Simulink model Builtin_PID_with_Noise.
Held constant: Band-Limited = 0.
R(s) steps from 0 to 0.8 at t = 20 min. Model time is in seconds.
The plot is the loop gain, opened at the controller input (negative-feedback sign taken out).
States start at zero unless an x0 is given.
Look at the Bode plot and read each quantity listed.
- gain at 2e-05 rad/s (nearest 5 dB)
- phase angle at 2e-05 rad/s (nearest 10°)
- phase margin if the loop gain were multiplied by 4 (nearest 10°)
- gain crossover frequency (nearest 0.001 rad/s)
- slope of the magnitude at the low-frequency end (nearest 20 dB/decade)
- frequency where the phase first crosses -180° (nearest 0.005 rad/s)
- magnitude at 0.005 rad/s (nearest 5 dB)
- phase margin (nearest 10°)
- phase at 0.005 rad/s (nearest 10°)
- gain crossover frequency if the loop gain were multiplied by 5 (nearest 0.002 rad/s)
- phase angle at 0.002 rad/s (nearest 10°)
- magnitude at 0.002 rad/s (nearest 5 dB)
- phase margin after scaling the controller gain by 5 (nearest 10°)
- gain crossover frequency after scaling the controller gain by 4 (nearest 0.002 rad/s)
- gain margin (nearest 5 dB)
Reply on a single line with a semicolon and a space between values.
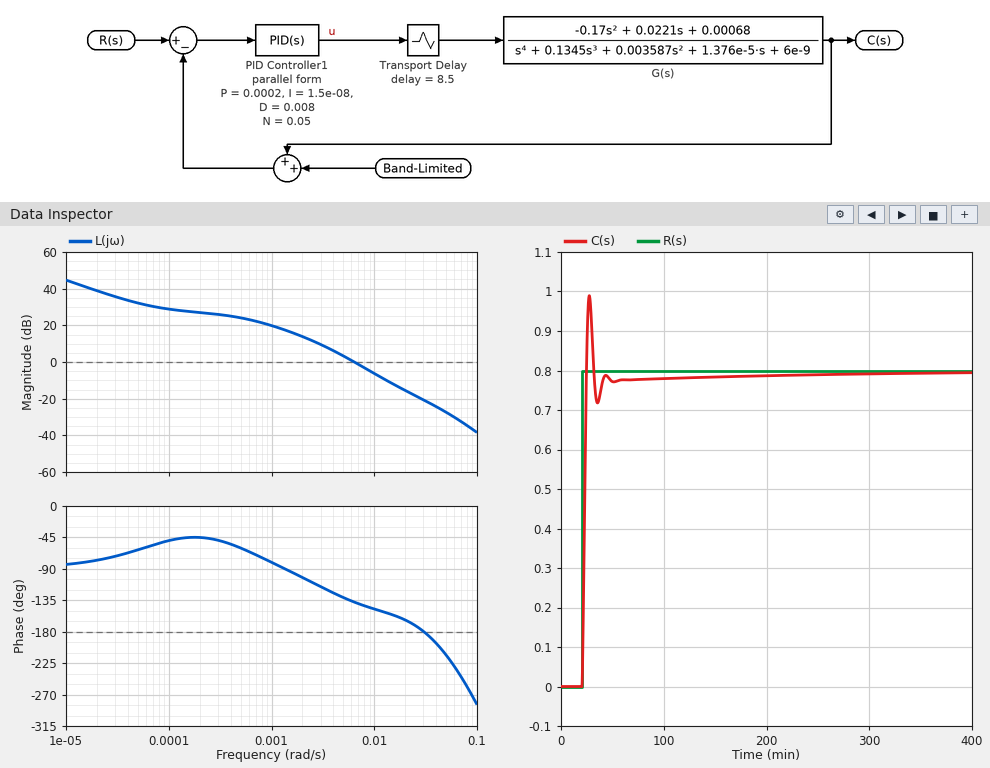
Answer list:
40 dB; -80°; 20°; 0.006 rad/s; -20 dB/decade; 0.030 rad/s; 5 dB; 40°; -130°; 0.018 rad/s; -100°; 15 dB; 20°; 0.016 rad/s; 20 dB
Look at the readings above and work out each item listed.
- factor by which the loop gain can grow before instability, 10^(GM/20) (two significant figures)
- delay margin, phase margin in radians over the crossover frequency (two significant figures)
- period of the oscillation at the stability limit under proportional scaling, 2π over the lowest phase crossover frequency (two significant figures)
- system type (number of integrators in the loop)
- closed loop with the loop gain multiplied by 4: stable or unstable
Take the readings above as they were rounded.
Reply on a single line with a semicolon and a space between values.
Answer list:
10; 120 s; 210 s; 1; stable
